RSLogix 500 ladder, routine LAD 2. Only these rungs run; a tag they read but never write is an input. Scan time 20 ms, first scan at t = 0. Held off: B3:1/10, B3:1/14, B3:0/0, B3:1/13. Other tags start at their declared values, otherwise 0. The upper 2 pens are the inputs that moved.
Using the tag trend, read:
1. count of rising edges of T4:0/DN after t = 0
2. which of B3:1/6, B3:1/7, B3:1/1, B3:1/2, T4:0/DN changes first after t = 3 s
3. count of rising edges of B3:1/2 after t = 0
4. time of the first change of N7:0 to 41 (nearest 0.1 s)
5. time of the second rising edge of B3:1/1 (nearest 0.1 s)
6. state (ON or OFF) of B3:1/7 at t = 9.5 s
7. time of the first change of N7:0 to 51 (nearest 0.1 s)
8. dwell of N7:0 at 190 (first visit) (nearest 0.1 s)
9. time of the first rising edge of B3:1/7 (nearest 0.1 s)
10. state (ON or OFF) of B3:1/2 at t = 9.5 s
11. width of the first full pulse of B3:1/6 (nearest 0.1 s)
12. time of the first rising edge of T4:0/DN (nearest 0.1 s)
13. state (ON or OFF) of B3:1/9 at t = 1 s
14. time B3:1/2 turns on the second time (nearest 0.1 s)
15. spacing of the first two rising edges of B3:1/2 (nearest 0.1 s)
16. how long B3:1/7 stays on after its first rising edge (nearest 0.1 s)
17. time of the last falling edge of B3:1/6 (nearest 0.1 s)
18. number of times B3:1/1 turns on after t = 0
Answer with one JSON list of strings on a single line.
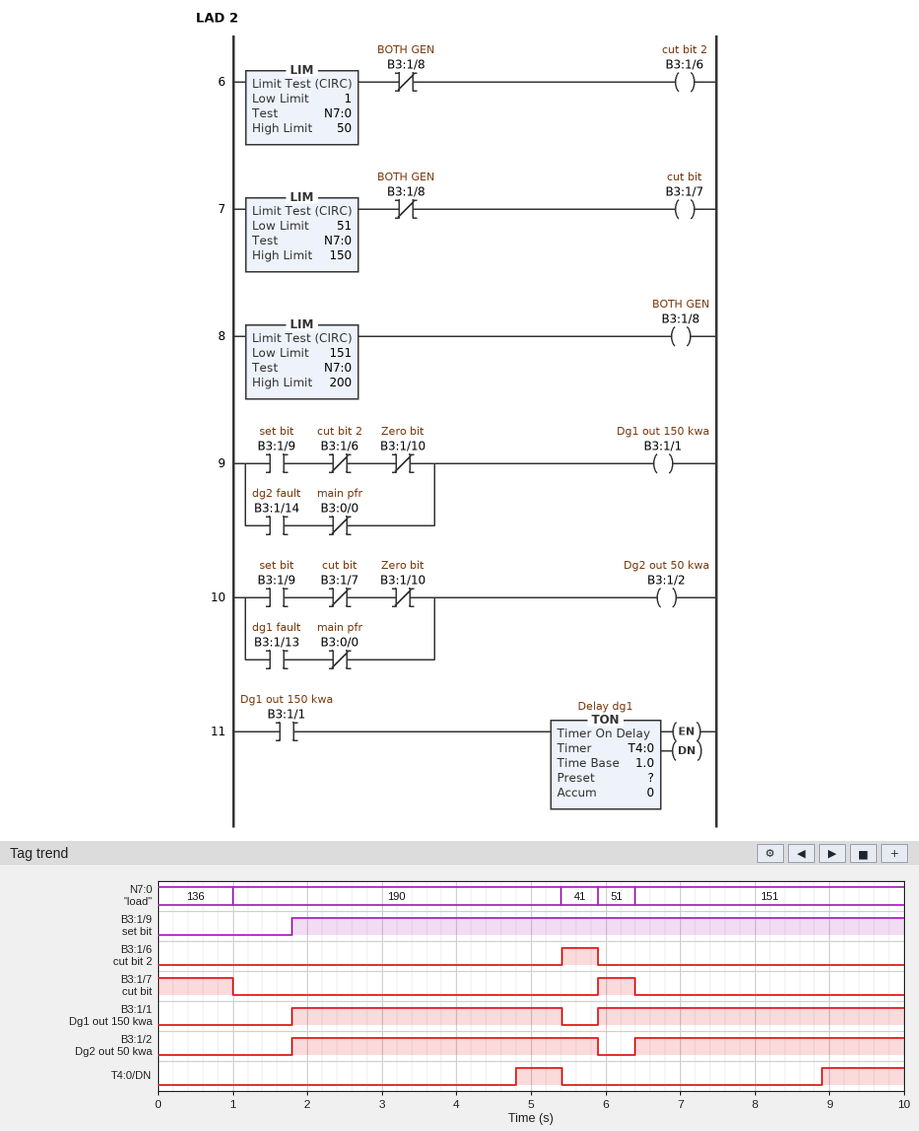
["2", "T4:0/DN", "2", "5.4 s", "5.9 s", "OFF", "5.9 s", "4.4 s", "5.9 s", "ON", "0.5 s", "4.8 s", "OFF", "6.4 s", "4.6 s", "0.5 s", "5.9 s", "2"]
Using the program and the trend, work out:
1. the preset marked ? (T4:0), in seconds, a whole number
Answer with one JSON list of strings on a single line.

["3 s"]
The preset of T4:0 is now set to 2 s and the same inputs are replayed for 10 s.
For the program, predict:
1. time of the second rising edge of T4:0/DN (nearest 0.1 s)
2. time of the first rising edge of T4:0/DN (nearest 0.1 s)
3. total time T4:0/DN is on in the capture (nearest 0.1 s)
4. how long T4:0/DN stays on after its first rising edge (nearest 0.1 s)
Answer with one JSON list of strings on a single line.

["7.9 s", "3.8 s", "3.7 s", "1.6 s"]
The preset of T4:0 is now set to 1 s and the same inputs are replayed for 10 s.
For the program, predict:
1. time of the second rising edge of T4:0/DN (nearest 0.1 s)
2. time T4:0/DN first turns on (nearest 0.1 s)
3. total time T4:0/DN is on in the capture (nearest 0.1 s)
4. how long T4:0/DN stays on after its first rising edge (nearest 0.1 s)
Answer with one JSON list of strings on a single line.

["6.9 s", "2.8 s", "5.7 s", "2.6 s"]
